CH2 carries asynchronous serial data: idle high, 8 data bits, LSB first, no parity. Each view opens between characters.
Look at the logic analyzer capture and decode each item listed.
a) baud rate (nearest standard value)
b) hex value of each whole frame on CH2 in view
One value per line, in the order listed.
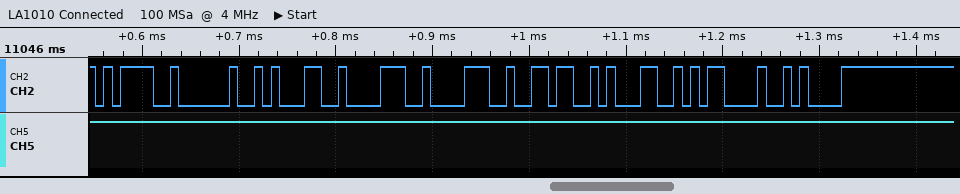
115200 baud
3D, 20, 31, 38, 38, 36, 31, 0D, 0A
